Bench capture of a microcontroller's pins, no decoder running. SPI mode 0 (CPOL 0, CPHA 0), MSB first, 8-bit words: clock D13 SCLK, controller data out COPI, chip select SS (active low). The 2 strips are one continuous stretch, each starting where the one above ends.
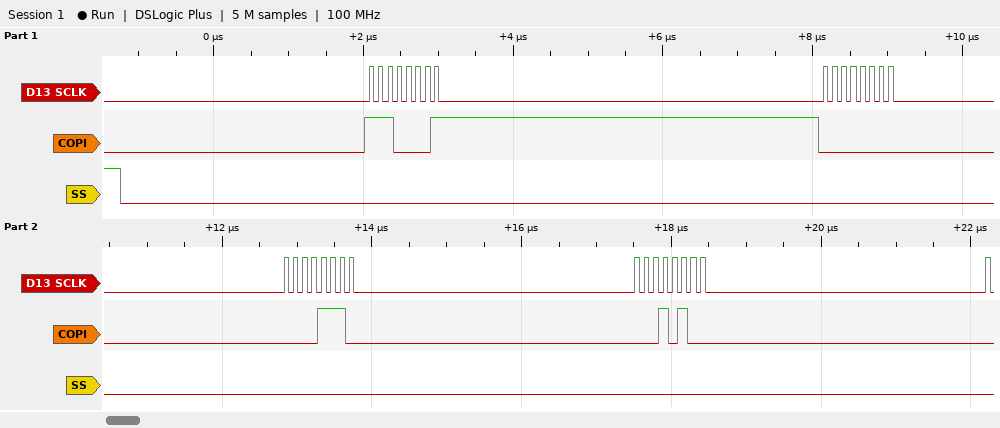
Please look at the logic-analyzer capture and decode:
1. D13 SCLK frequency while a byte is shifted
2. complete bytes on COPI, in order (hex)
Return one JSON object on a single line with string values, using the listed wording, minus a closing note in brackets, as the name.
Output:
{"D13 SCLK frequency while a byte is shifted": "8 MHz", "complete bytes on COPI, in order": "0xE1 0x00 0x0E 0x14"}
